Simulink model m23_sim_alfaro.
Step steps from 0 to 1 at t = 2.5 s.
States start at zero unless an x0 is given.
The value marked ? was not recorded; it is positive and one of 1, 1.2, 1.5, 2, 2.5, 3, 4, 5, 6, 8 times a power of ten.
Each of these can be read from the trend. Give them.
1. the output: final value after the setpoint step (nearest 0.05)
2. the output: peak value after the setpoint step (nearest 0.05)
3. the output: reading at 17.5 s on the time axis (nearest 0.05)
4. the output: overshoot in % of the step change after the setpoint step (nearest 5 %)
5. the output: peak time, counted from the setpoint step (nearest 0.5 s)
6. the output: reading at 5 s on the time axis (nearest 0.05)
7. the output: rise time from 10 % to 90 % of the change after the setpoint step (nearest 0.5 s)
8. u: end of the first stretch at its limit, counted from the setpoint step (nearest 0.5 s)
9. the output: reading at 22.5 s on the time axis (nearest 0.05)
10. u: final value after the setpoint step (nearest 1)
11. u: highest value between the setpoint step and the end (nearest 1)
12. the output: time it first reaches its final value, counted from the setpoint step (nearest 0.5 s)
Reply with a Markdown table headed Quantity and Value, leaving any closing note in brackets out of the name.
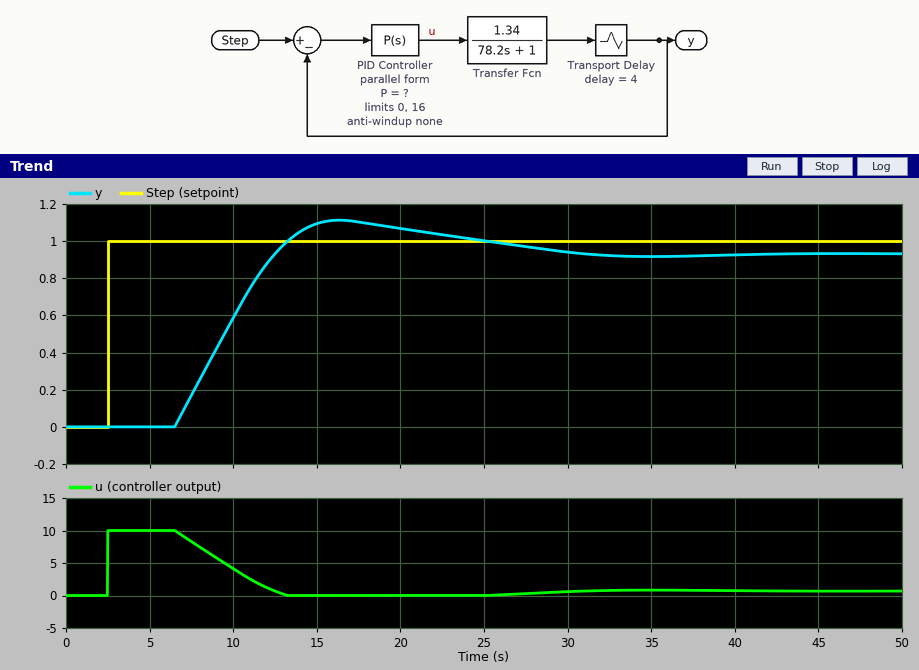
| Quantity | Value |
|---|---|
| the output: final value after the setpoint step | 0.95 |
| the output: peak value after the setpoint step | 1.10 |
| the output: reading at 17.5 s on the time axis | 1.10 |
| the output: overshoot in % of the step change after the setpoint step | 20 % |
| the output: peak time, counted from the setpoint step | 14.0 s |
| the output: reading at 5 s on the time axis | 0.00 |
| the output: rise time from 10 % to 90 % of the change after the setpoint step | 4.5 s |
| u: end of the first stretch at its limit, counted from the setpoint step | 4.0 s |
| the output: reading at 22.5 s on the time axis | 1.05 |
| u: final value after the setpoint step | 1 |
| u: highest value between the setpoint step and the end | 10 |
| the output: time it first reaches its final value, counted from the setpoint step | 10.0 s |
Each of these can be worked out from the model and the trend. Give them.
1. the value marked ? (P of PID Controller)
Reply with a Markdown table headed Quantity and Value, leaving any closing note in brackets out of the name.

| Quantity | Value |
|---|---|
| the value marked ? | 10 |
